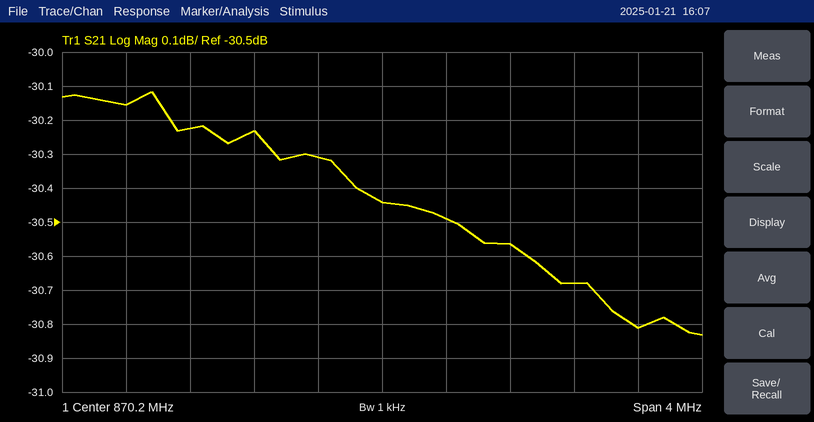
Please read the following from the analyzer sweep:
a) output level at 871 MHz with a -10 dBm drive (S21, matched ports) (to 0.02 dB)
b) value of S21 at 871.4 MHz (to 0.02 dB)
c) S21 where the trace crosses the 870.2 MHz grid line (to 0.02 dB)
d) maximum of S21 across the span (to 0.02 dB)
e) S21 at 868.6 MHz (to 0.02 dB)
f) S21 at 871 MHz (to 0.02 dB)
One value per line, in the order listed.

-40.56 dBm
-30.68 dB
-30.44 dB
-30.12 dB
-30.16 dB
-30.56 dB
